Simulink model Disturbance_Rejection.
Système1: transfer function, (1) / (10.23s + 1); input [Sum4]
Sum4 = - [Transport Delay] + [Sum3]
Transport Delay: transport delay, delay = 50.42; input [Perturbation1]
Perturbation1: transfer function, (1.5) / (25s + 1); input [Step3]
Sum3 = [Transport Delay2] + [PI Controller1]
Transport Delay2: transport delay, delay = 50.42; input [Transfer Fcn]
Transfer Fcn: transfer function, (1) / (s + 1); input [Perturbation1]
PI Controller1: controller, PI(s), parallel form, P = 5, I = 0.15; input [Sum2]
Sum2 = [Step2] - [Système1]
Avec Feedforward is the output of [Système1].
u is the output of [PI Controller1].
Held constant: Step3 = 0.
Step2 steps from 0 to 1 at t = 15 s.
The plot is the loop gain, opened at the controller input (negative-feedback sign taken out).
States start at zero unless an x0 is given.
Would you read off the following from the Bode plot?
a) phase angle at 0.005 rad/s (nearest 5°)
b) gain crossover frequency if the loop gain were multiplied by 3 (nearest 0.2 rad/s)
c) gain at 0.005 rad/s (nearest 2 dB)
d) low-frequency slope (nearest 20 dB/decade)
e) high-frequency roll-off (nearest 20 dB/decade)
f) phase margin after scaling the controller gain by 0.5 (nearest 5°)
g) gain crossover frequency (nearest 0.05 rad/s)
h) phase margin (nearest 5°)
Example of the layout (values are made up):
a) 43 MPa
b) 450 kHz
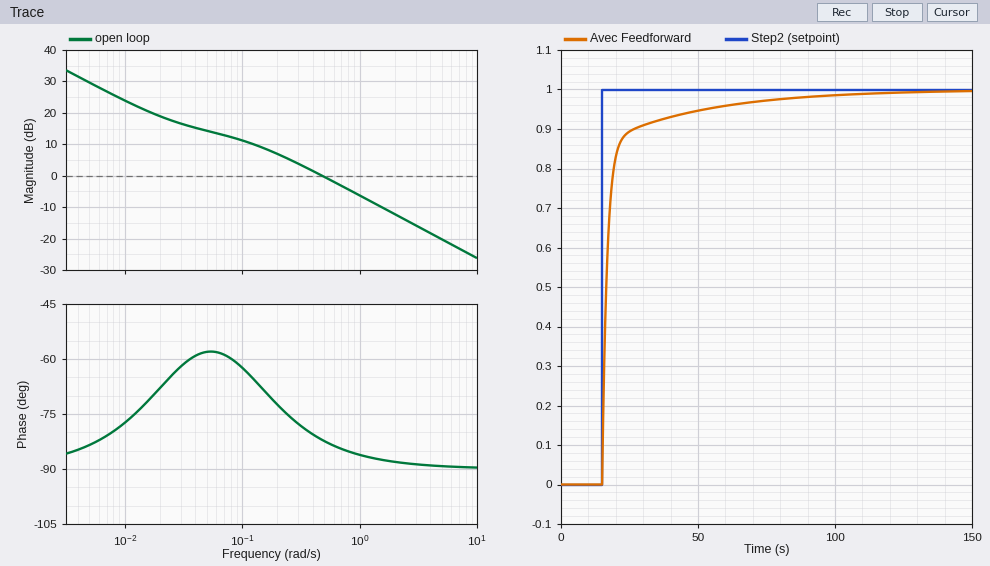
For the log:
a) -85°
b) 1.4 rad/s
c) 30 dB
d) -20 dB/decade
e) -20 dB/decade
f) 105°
g) 0.50 rad/s
h) 100°
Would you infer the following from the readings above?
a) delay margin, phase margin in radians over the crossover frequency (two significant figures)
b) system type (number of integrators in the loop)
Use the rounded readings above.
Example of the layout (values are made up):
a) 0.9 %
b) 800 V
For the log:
a) 3.5 s
b) 1
